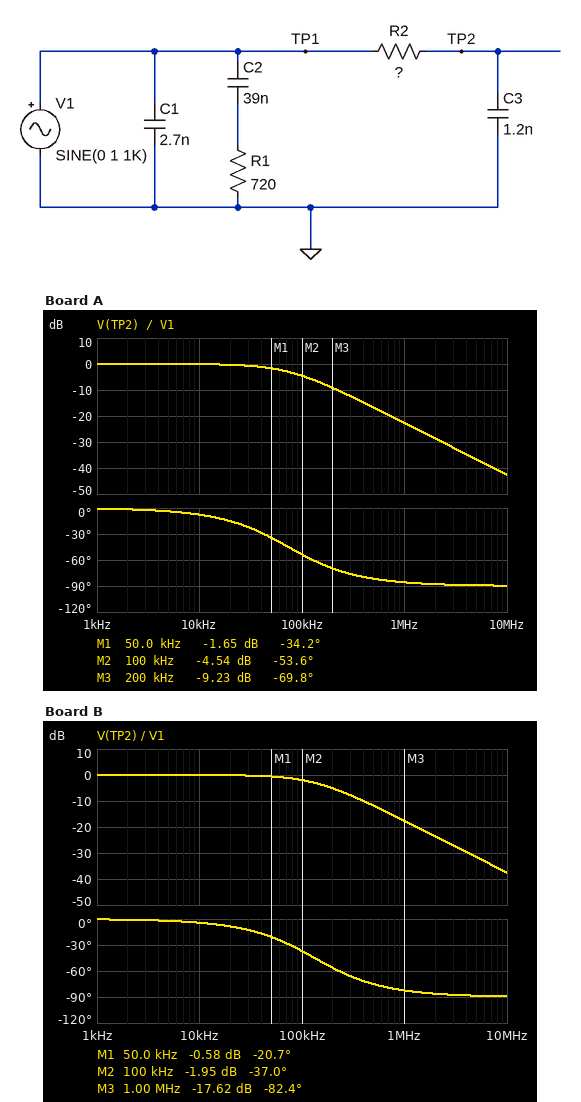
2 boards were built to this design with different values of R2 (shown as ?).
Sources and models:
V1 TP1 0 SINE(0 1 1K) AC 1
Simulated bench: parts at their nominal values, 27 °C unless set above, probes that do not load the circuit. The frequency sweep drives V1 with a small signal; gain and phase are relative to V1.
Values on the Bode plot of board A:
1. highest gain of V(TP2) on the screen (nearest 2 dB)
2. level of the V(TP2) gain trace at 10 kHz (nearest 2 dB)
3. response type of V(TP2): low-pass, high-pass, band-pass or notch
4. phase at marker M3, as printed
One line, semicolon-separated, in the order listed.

0 dB; 0 dB; low-pass; -69.8 deg
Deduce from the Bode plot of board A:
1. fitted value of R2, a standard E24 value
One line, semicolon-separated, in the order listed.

1.8 kΩ
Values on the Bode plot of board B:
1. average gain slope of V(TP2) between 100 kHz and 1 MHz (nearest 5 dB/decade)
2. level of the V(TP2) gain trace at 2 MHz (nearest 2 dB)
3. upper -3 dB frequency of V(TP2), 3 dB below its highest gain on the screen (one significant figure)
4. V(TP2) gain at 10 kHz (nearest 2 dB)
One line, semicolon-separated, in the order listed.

-15 dB/decade; -24 dB; 100 kHz; 0 dB
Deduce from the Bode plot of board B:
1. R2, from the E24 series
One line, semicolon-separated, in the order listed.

1 kΩ
